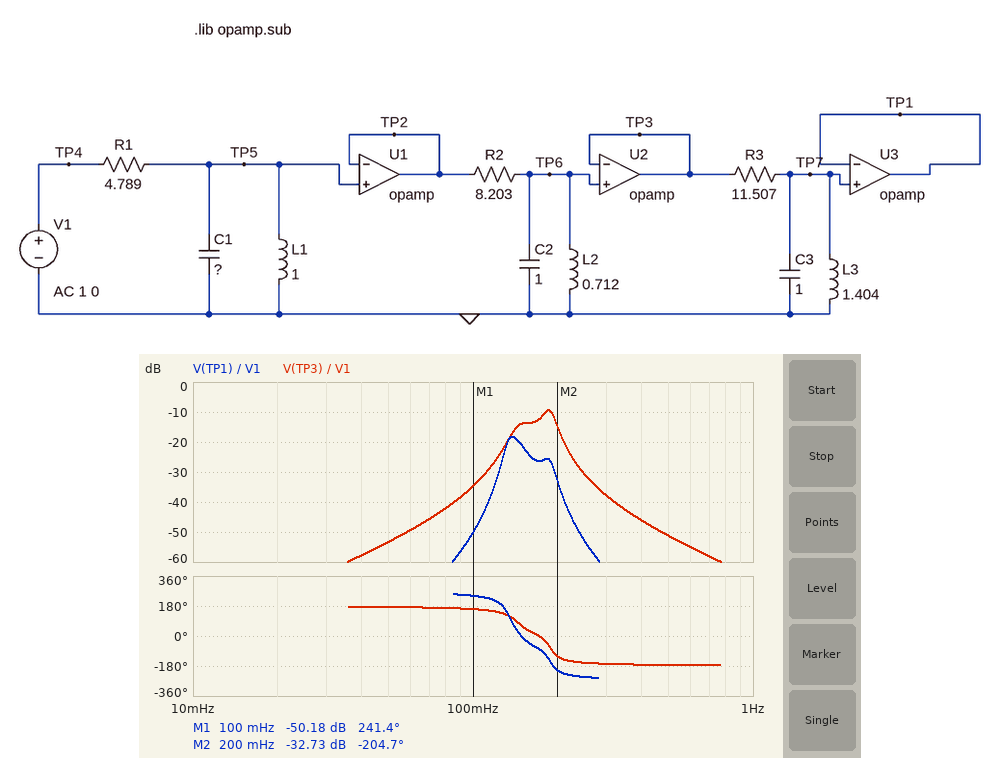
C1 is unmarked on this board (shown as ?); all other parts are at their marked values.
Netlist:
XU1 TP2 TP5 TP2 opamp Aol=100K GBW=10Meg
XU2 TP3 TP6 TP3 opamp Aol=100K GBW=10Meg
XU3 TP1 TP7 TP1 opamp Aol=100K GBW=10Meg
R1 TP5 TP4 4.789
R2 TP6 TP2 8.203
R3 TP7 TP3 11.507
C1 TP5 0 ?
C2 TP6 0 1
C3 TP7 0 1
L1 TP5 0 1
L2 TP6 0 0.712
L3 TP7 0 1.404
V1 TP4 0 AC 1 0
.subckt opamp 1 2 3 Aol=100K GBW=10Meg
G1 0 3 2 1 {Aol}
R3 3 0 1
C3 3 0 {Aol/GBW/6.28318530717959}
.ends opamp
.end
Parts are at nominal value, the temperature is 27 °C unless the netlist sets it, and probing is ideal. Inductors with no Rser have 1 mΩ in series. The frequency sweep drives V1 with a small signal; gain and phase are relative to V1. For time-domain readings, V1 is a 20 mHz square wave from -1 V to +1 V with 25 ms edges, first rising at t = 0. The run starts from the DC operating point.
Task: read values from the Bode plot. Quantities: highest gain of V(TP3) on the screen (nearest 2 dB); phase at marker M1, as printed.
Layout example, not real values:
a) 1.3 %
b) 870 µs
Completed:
a) -10 dB
b) 241.4 deg
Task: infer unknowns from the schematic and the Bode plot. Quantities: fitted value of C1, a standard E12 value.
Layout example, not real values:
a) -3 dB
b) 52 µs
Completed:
a) 1.2 F
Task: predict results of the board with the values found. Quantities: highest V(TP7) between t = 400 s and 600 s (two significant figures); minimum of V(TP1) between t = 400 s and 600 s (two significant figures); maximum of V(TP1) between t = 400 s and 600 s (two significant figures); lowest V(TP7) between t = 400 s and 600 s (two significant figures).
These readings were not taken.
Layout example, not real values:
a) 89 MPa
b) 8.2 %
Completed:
a) 30 mV
b) -30 mV
c) 30 mV
d) -30 mV
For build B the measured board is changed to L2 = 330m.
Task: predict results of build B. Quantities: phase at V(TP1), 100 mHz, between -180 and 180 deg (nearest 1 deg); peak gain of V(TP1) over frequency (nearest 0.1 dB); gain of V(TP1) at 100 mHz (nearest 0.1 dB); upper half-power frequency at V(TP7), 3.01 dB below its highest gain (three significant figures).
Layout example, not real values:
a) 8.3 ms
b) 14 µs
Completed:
a) -116 deg
b) -28.9 dB
c) -58.5 dB
d) 147 mHz
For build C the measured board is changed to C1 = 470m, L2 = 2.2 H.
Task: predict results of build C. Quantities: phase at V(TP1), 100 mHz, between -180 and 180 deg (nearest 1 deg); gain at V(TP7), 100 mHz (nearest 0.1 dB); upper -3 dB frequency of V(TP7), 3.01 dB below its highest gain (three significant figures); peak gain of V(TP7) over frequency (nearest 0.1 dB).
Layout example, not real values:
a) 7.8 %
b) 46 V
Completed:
a) -161 deg
b) -33.5 dB
c) 140 mHz
d) -20.5 dB
